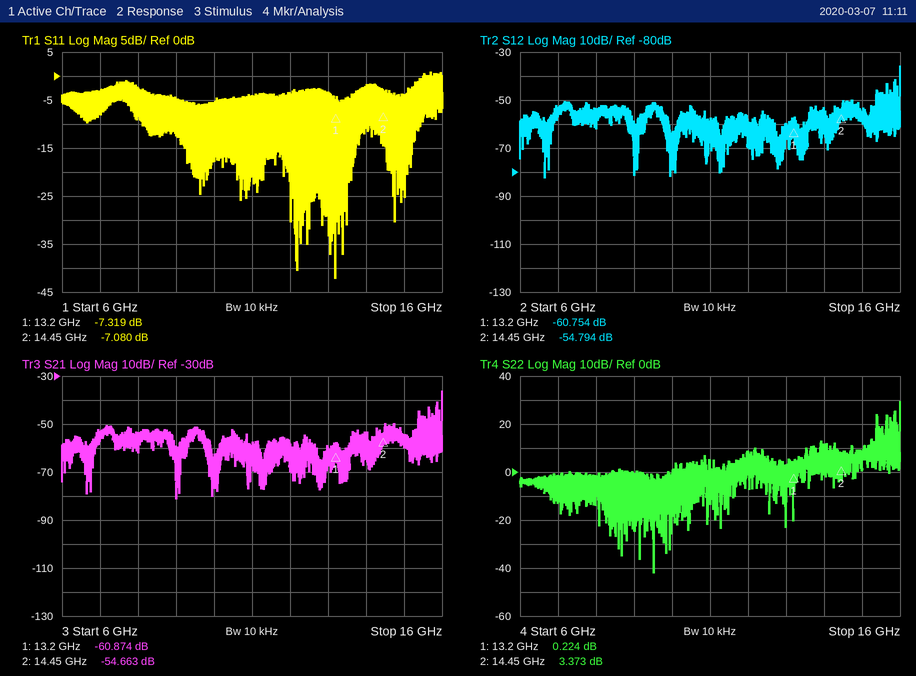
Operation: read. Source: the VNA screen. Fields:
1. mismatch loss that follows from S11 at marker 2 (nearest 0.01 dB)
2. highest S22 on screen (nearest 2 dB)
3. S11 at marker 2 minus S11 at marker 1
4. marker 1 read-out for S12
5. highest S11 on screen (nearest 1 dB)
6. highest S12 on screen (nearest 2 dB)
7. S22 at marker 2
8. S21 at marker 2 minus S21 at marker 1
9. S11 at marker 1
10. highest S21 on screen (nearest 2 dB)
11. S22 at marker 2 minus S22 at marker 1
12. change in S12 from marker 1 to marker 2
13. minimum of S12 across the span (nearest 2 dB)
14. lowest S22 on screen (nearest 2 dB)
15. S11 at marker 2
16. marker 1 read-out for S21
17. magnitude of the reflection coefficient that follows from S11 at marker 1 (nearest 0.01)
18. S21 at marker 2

0.95 dB
30 dB
0.239 dB
-60.754 dB
1 dB
-36 dB
3.373 dB
6.211 dB
-7.319 dB
-36 dB
3.149 dB
5.960 dB
-82 dB
-42 dB
-7.080 dB
-60.874 dB
0.43
-54.663 dB
